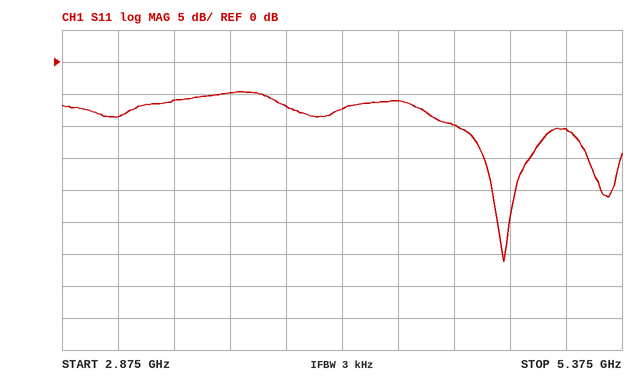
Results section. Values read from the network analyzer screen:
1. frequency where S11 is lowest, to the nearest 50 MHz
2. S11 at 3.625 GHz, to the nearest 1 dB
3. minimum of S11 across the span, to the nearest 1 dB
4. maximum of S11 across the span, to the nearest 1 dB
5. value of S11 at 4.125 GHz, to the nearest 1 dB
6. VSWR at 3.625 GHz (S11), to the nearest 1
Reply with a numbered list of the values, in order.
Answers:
1. 4.85 GHz
2. -5 dB
3. -31 dB
4. -5 dB
5. -7 dB
6. 4
